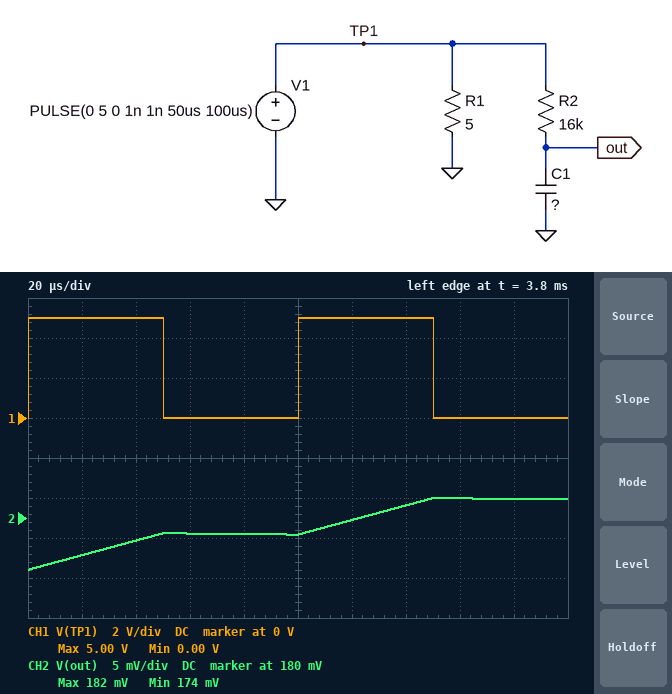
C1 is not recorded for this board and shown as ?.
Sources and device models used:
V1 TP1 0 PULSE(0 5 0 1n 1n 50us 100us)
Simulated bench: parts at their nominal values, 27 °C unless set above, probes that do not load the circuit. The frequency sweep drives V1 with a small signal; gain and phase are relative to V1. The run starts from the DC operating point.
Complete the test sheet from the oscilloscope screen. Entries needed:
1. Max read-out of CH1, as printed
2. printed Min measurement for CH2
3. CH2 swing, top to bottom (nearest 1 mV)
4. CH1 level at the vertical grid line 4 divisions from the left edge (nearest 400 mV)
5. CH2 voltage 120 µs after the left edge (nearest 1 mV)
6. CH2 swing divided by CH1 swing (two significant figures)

5.00 V
174 mV
9 mV
0 V
180 mV
0.0018
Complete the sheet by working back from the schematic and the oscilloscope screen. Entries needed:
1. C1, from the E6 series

3.3 µF
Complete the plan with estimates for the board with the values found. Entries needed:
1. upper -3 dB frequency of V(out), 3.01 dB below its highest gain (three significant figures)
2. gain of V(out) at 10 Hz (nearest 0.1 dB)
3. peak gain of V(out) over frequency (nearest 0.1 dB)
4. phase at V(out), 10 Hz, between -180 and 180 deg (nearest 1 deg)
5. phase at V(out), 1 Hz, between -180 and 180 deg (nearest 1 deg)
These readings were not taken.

3.01 Hz
-10.8 dB
0 dB
-73 deg
-18 deg
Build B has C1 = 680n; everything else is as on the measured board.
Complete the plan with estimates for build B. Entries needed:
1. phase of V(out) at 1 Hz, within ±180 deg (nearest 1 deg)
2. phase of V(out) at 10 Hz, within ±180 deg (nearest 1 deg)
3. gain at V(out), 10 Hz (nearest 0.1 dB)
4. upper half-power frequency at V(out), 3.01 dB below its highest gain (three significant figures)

-4 deg
-34 deg
-1.7 dB
14.6 Hz
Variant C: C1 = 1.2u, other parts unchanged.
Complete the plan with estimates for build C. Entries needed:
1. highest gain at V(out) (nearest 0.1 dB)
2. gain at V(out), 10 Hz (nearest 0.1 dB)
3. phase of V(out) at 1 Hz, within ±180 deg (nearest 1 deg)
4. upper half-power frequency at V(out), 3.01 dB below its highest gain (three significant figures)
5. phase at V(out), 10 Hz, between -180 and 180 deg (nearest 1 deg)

0 dB
-3.9 dB
-7 deg
8.29 Hz
-50 deg
